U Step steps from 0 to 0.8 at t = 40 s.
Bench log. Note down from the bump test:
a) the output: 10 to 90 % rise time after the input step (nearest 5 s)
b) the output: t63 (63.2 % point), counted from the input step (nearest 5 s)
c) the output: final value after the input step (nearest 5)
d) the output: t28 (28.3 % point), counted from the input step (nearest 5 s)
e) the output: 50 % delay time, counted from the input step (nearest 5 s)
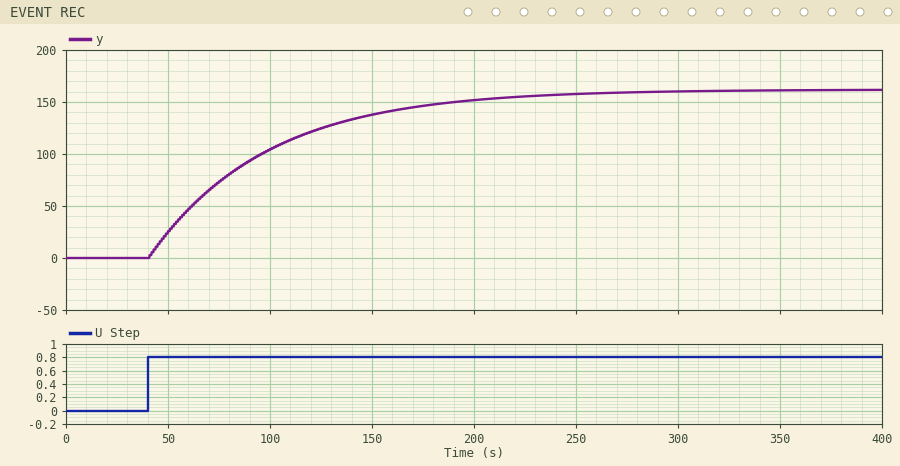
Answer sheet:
125 s
60 s
160
20 s
40 s
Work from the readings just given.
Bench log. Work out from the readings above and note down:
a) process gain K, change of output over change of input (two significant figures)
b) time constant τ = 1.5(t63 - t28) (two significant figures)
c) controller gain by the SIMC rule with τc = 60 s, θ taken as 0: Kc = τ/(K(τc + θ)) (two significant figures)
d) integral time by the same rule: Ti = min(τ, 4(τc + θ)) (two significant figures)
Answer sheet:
200
60 s
0.0050
60 s
